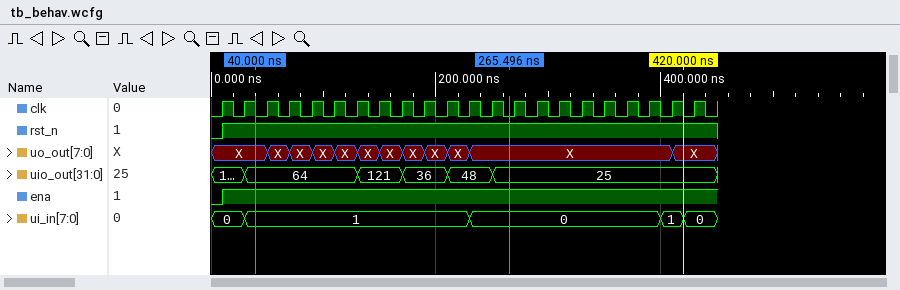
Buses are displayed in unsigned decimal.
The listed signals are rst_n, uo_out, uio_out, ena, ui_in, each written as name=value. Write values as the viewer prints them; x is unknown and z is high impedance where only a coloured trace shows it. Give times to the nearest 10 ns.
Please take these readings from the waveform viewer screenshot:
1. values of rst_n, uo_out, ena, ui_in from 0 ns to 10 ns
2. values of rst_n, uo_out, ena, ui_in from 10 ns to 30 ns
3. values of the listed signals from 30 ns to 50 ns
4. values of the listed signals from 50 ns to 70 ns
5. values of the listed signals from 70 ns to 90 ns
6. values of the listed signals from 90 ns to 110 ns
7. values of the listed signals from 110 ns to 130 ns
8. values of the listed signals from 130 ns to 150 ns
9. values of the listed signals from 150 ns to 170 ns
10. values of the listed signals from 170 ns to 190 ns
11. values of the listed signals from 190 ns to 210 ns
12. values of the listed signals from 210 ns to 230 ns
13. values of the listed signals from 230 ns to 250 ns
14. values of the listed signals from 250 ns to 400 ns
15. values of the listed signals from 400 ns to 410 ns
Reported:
rst_n=0, uo_out=X, ena=0, ui_in=0
rst_n=1, uo_out=X, ena=1, ui_in=0
rst_n=1, uo_out=X, uio_out=64, ena=1, ui_in=1
rst_n=1, uo_out=X, uio_out=64, ena=1, ui_in=1
rst_n=1, uo_out=X, uio_out=64, ena=1, ui_in=1
rst_n=1, uo_out=X, uio_out=64, ena=1, ui_in=1
rst_n=1, uo_out=X, uio_out=64, ena=1, ui_in=1
rst_n=1, uo_out=X, uio_out=121, ena=1, ui_in=1
rst_n=1, uo_out=X, uio_out=121, ena=1, ui_in=1
rst_n=1, uo_out=X, uio_out=36, ena=1, ui_in=1
rst_n=1, uo_out=X, uio_out=36, ena=1, ui_in=1
rst_n=1, uo_out=X, uio_out=48, ena=1, ui_in=1
rst_n=1, uo_out=X, uio_out=48, ena=1, ui_in=0
rst_n=1, uo_out=X, uio_out=25, ena=1, ui_in=0
rst_n=1, uo_out=X, uio_out=25, ena=1, ui_in=1
